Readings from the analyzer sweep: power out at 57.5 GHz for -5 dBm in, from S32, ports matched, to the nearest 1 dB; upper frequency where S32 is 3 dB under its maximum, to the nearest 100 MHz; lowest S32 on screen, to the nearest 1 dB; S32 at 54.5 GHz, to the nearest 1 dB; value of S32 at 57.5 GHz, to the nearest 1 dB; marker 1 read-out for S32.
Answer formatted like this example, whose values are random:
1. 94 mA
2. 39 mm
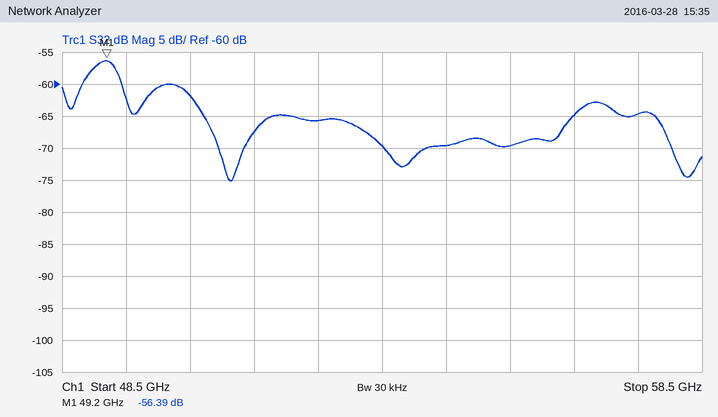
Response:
1. -70 dBm
2. 49.4 GHz
3. -75 dB
4. -70 dB
5. -65 dB
6. -56.39 dB
